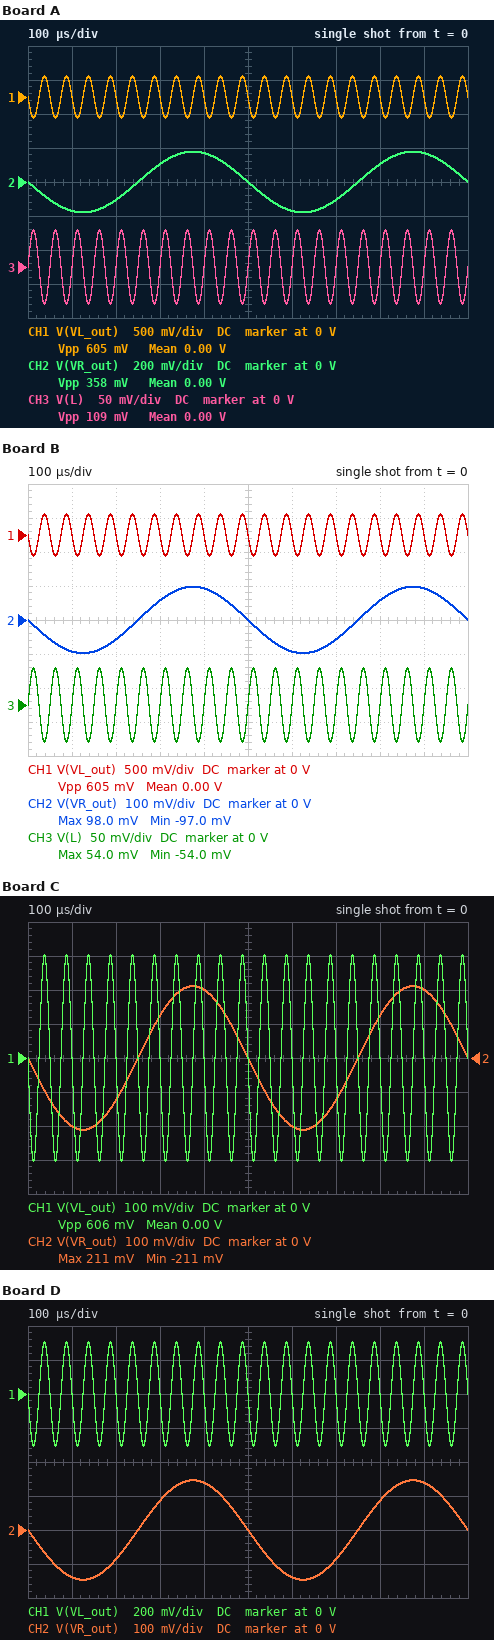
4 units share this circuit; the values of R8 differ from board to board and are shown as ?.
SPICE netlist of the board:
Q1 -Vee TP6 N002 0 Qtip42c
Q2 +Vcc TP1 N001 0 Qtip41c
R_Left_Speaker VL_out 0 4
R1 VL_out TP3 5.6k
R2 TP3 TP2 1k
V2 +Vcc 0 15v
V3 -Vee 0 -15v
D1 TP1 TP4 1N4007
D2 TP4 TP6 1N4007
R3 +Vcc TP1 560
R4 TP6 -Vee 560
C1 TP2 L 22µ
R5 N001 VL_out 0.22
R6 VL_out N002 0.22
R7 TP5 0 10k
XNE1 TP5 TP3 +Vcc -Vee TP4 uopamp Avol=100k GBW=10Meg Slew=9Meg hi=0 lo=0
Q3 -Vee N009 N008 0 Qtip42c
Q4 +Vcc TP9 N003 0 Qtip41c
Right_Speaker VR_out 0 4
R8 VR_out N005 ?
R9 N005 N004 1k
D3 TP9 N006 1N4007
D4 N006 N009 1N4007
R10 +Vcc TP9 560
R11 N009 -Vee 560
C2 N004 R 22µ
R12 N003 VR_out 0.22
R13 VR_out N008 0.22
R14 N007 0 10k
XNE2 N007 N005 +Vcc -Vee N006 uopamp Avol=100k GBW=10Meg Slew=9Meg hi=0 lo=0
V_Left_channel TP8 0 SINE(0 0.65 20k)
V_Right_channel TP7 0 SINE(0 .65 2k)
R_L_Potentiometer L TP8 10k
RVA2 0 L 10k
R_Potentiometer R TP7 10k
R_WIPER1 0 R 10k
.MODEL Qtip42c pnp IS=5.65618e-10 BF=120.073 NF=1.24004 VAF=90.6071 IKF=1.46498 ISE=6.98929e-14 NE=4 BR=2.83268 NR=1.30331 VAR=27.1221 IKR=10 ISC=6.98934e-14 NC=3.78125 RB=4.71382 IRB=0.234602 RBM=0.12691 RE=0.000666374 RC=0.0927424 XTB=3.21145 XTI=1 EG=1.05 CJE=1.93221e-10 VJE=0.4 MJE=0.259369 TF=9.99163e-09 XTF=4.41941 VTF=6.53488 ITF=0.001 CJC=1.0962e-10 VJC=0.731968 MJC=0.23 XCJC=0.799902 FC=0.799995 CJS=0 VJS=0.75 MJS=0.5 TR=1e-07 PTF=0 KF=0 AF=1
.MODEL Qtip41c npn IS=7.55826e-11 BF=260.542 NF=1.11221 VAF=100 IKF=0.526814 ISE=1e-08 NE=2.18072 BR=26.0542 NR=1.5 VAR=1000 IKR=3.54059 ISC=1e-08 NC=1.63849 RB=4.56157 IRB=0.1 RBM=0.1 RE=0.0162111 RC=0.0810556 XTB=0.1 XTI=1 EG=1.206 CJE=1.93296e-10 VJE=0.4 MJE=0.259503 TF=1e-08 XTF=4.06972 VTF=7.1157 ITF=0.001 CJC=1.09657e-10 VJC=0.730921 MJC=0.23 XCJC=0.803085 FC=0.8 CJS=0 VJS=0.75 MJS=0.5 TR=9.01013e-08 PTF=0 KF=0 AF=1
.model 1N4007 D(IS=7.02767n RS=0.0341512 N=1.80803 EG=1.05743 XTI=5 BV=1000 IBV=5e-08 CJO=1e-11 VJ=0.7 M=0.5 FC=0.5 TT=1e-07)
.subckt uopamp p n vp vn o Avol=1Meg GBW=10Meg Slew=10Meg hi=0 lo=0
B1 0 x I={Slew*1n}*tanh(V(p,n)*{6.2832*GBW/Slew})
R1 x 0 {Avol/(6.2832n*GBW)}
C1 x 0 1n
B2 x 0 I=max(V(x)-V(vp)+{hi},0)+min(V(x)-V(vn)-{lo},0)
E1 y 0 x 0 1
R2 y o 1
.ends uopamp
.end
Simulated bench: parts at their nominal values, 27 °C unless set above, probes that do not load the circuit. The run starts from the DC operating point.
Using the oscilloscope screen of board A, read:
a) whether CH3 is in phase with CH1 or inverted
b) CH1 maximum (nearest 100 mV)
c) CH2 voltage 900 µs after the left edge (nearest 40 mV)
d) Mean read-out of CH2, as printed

inverted
300 mV
160 mV
0.00 V
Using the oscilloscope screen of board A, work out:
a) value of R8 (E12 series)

3.3 kΩ
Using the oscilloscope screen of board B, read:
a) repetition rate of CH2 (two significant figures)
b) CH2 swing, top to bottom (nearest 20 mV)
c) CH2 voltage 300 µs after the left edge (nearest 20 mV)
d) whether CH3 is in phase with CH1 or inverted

2.0 kHz
200 mV
60 mV
inverted
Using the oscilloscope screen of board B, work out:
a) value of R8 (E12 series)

1.8 kΩ
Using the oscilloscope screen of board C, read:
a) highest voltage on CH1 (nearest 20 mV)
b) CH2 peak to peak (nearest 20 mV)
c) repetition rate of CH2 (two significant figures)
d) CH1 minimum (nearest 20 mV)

300 mV
420 mV
2.0 kHz
-300 mV
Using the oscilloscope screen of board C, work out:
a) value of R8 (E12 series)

3.9 kΩ
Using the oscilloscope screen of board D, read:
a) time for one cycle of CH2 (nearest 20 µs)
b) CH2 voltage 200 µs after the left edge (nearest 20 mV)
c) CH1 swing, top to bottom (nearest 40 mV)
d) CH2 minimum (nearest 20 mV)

500 µs
-80 mV
600 mV
-140 mV
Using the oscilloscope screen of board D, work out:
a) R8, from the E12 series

2.7 kΩ
